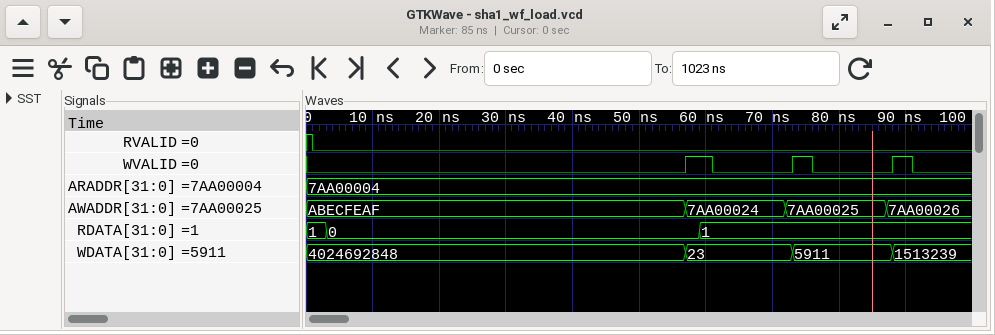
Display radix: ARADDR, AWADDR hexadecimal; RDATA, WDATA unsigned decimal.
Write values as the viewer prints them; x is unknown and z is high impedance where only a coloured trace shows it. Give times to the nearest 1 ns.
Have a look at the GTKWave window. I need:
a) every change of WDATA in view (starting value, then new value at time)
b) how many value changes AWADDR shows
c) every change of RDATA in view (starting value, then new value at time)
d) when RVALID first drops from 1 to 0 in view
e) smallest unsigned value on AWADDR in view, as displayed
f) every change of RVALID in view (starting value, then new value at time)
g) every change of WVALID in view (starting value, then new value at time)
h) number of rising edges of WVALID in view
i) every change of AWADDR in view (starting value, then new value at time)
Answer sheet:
4024692848, 23 at 57 ns, 5911 at 73 ns, 1513239 at 88 ns
3
1, 0 at 3 ns, 1 at 59 ns
1 ns
7AA00024
1, 0 at 1 ns
0, 1 at 57 ns, 0 at 61 ns, 1 at 73 ns, 0 at 76 ns, 1 at 88 ns, 0 at 91 ns
3
ABECFEAF, 7AA00024 at 57 ns, 7AA00025 at 72 ns, 7AA00026 at 87 ns
